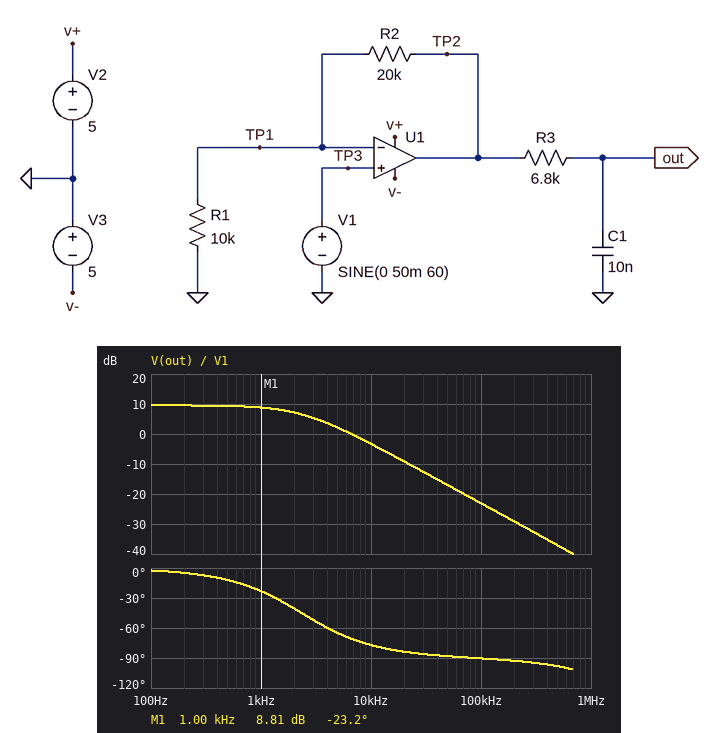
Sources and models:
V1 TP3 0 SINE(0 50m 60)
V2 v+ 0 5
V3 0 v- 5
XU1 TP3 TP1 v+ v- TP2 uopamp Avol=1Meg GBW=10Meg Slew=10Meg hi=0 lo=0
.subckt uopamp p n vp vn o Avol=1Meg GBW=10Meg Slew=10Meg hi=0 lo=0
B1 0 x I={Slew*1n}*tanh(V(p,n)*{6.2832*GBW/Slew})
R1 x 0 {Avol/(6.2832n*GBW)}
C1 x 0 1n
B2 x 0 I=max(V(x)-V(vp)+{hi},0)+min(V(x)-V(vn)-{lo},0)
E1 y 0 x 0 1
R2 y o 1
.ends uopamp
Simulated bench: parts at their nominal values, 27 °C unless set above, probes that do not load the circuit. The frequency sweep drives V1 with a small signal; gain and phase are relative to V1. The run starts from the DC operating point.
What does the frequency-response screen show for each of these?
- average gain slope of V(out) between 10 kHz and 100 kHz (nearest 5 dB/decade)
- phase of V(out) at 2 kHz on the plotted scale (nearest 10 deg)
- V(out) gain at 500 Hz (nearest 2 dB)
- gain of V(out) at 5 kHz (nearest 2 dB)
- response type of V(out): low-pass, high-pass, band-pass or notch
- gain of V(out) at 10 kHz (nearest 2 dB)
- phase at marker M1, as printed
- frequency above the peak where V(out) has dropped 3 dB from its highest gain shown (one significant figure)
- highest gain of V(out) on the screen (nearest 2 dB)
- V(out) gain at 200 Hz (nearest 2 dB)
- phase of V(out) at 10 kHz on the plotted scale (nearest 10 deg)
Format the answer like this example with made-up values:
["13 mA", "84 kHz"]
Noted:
["-20 dB/decade", "-40 deg", "10 dB", "2 dB", "low-pass", "-4 dB", "-23.2 deg", "2 kHz", "10 dB", "10 dB", "-80 deg"]
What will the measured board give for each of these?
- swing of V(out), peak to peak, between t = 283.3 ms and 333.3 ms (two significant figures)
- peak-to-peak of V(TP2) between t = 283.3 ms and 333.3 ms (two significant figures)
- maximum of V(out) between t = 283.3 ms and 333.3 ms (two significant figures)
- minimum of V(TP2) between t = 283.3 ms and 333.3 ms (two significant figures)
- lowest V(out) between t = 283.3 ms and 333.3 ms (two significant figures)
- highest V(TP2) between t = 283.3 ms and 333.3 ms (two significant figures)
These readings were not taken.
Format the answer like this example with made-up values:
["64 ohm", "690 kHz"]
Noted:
["300 mV", "300 mV", "150 mV", "-150 mV", "-150 mV", "150 mV"]
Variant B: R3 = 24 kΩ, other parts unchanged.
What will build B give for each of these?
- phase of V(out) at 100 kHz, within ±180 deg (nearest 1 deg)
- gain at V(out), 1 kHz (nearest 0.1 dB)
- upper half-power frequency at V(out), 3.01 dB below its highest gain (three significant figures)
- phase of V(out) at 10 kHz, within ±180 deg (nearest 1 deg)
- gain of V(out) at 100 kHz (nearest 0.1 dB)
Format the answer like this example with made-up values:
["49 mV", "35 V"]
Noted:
["-91 deg", "4.4 dB", "663 Hz", "-86 deg", "-34.0 dB"]
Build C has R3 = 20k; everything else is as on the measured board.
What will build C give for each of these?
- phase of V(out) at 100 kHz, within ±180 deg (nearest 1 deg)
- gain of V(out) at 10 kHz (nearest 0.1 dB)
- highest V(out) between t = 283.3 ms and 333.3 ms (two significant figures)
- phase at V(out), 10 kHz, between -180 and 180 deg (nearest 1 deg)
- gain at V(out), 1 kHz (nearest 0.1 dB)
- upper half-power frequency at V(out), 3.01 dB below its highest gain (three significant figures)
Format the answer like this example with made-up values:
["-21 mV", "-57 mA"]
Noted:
["-91 deg", "-12.5 dB", "150 mV", "-86 deg", "5.4 dB", "796 Hz"]
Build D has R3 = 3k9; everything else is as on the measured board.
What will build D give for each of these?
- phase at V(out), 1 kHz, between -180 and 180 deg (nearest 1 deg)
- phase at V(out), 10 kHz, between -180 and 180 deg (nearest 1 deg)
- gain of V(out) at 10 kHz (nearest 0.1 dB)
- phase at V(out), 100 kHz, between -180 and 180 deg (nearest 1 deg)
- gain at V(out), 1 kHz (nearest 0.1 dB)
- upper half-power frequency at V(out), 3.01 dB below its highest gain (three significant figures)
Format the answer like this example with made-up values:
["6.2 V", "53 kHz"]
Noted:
["-14 deg", "-68 deg", "1.1 dB", "-89 deg", "9.3 dB", "4.08 kHz"]
